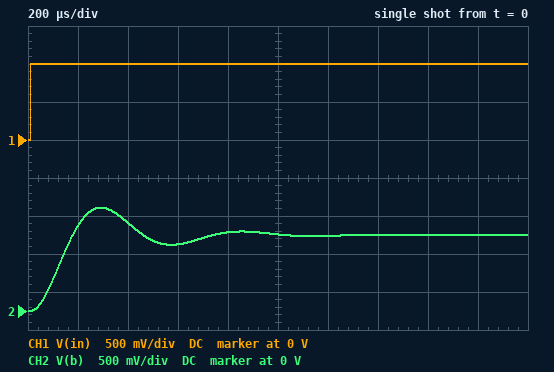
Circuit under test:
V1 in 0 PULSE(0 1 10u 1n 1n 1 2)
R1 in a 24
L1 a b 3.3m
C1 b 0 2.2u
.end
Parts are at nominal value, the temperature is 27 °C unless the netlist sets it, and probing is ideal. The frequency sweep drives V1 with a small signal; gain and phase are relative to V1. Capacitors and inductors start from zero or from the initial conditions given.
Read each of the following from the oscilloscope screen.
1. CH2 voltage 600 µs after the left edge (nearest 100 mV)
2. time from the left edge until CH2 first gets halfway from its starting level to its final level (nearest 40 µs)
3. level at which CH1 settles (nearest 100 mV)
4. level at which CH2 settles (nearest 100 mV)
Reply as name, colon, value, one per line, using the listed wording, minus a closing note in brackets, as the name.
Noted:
CH2 voltage 600 µs after the left edge: 900 mV
time from the left edge until CH2 first gets halfway from its starting level to its final level: 120 µs
level at which CH1 settles: 1.0 V
level at which CH2 settles: 1.0 V
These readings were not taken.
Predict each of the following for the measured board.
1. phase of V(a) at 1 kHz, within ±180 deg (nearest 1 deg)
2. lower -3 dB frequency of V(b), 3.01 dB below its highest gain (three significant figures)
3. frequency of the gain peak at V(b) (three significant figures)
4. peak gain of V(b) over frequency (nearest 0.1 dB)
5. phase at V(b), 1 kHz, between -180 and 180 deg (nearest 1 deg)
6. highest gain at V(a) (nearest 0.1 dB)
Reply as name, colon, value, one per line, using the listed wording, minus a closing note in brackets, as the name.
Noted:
phase of V(a) at 1 kHz, within ±180 deg: -25 deg
lower -3 dB frequency of V(b), 3.01 dB below its highest gain: 874 Hz
frequency of the gain peak at V(b): 1.68 kHz
peak gain of V(b) over frequency: 4.6 dB
phase at V(b), 1 kHz, between -180 and 180 deg: -25 deg
highest gain at V(a): 0 dB
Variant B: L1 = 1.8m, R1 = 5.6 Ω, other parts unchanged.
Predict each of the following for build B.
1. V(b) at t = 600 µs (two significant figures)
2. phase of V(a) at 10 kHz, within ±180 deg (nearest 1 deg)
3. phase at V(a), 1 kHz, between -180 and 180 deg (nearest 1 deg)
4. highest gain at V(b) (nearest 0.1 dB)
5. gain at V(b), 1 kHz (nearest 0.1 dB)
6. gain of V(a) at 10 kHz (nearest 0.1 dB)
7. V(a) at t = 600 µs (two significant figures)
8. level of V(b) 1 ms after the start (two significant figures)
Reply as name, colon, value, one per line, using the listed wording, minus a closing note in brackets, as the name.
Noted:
V(b) at t = 600 µs: 1.4 V
phase of V(a) at 10 kHz, within ±180 deg: 3 deg
phase at V(a), 1 kHz, between -180 and 180 deg: -5 deg
highest gain at V(b): 14.2 dB
gain at V(b), 1 kHz: 1.4 dB
gain of V(a) at 10 kHz: 0 dB
V(a) at t = 600 µs: 990 mV
level of V(b) 1 ms after the start: 1.2 V
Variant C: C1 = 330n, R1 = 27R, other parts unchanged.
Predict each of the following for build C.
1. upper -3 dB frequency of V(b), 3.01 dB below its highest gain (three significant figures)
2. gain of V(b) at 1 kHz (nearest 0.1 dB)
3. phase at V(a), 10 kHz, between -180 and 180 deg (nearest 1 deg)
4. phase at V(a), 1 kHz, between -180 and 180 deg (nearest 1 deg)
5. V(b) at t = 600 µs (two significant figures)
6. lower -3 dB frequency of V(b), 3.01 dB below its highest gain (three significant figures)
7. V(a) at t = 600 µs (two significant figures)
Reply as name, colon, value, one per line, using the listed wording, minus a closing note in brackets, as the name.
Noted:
upper -3 dB frequency of V(b), 3.01 dB below its highest gain: 5.35 kHz
gain of V(b) at 1 kHz: 0.4 dB
phase at V(a), 10 kHz, between -180 and 180 deg: 10 deg
phase at V(a), 1 kHz, between -180 and 180 deg: -3 deg
V(b) at t = 600 µs: 970 mV
lower -3 dB frequency of V(b), 3.01 dB below its highest gain: 4.02 kHz
V(a) at t = 600 µs: 1.0 V
